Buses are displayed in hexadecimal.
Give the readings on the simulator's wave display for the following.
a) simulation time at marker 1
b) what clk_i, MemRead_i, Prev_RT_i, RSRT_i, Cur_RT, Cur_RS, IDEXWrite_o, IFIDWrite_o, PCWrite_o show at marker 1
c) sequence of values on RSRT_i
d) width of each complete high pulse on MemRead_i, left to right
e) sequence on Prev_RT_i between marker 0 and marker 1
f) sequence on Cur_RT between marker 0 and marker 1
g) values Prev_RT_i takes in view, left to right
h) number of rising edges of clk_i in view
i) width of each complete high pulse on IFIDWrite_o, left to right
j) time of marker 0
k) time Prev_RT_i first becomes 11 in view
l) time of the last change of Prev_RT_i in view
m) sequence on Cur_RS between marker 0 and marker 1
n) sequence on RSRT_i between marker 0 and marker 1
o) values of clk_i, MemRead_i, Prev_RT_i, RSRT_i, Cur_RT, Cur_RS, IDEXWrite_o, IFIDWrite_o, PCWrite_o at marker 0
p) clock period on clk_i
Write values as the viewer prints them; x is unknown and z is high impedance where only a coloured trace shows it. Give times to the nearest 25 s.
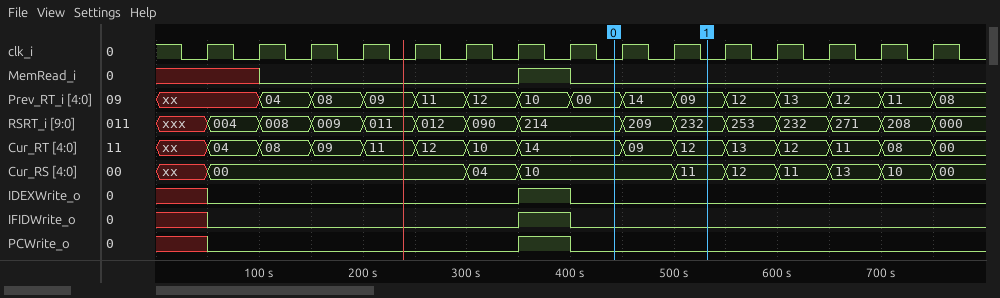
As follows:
525 s
clk_i=0, MemRead_i=0, Prev_RT_i=09, RSRT_i=232, Cur_RT=12, Cur_RS=11, IDEXWrite_o=0, IFIDWrite_o=0, PCWrite_o=0
xxx, 004, 008, 009, 011, 012, 090, 214, 209, 232, 253, 232, 271, 208, 000
50 s
00, 14, 09
14, 09, 12
xx, 04, 08, 09, 11, 12, 10, 00, 14, 09, 12, 13, 12, 11, 08
15
50 s
450 s
250 s
750 s
10, 11
214, 209, 232
clk_i=0, MemRead_i=0, Prev_RT_i=00, RSRT_i=214, Cur_RT=14, Cur_RS=10, IDEXWrite_o=0, IFIDWrite_o=0, PCWrite_o=0
50 s
